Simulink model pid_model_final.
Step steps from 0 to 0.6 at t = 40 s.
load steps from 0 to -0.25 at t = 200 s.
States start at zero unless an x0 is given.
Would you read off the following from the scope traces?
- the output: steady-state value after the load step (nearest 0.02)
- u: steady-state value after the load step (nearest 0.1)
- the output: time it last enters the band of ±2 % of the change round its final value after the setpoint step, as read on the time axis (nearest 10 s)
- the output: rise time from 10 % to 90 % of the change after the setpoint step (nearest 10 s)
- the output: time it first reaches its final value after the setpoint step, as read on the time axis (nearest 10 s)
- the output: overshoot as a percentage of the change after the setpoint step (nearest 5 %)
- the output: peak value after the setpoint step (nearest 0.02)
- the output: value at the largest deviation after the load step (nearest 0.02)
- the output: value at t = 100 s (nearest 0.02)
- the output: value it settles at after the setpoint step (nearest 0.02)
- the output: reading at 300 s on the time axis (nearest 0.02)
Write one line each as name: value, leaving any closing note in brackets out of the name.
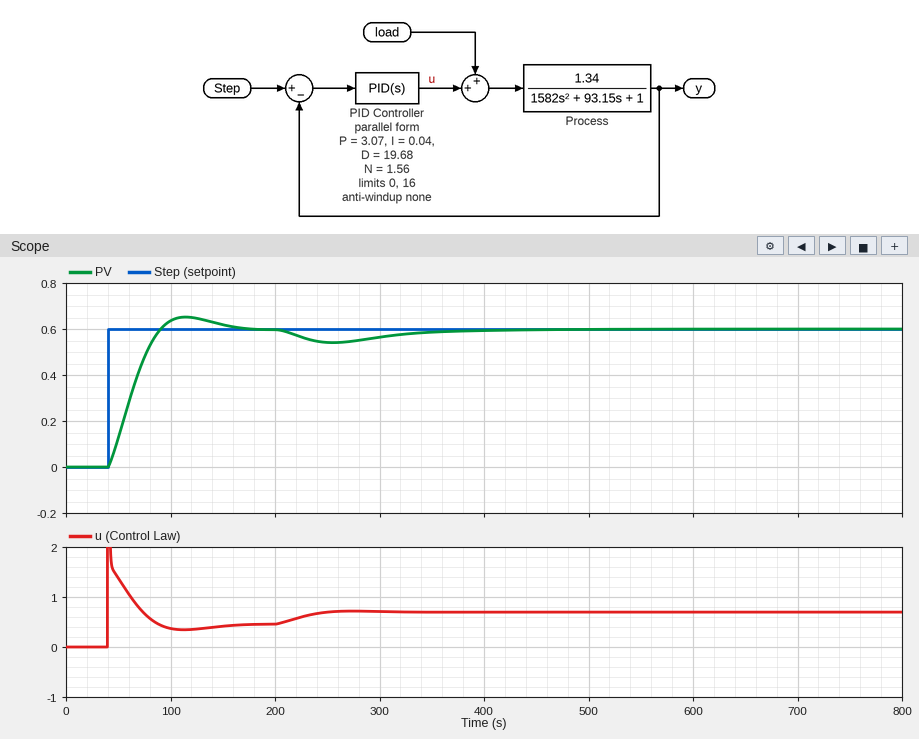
the output: steady-state value after the load step: 0.60
u: steady-state value after the load step: 0.7
the output: time it last enters the band of ±2 % of the change round its final value after the setpoint step, as read on the time axis: 160 s
the output: rise time from 10 % to 90 % of the change after the setpoint step: 40 s
the output: time it first reaches its final value after the setpoint step, as read on the time axis: 90 s
the output: overshoot as a percentage of the change after the setpoint step: 10 %
the output: peak value after the setpoint step: 0.66
the output: value at the largest deviation after the load step: 0.54
the output: value at t = 100 s: 0.64
the output: value it settles at after the setpoint step: 0.60
the output: reading at 300 s on the time axis: 0.56
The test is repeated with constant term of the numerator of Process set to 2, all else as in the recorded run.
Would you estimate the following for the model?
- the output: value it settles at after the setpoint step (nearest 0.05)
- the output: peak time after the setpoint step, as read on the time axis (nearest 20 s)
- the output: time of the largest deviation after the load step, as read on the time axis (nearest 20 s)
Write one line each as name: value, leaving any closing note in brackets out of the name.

the output: value it settles at after the setpoint step: 0.60
the output: peak time after the setpoint step, as read on the time axis: 100 s
the output: time of the largest deviation after the load step, as read on the time axis: 240 s
